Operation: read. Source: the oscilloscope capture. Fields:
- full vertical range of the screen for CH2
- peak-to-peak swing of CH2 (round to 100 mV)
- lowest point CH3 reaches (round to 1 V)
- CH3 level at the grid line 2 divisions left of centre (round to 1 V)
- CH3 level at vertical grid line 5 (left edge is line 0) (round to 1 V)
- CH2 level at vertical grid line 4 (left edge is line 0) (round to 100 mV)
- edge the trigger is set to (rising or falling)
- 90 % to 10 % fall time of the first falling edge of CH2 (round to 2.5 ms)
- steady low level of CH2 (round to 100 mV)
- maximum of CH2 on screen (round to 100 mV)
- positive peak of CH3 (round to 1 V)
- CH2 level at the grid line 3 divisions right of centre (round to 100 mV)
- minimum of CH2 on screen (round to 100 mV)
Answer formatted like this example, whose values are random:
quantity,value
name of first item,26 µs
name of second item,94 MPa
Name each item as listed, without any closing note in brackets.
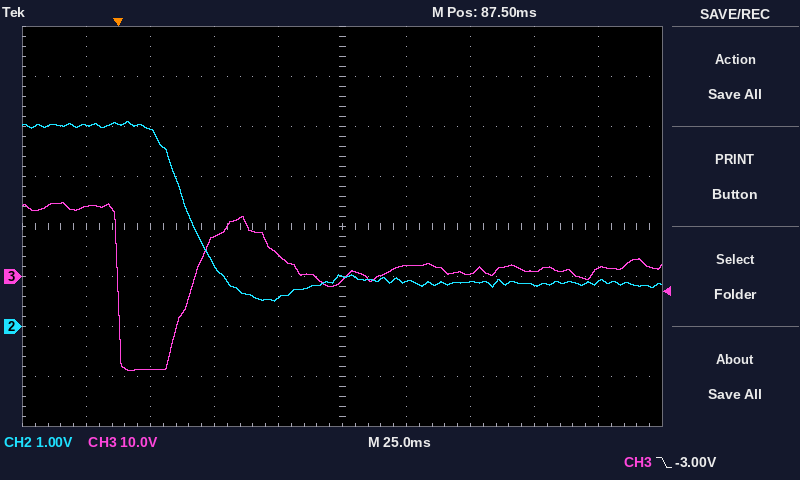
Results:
quantity,value
full vertical range of the screen for CH2,8 V
peak-to-peak swing of CH2,3.6 V
lowest point CH3 reaches,-19 V
CH3 level at the grid line 2 divisions left of centre,8 V
CH3 level at vertical grid line 5 (left edge is line 0),-1 V
CH2 level at vertical grid line 4 (left edge is line 0),600 mV
edge the trigger is set to,falling
90 % to 10 % fall time of the first falling edge of CH2,22.5 ms
steady low level of CH2,900 mV
maximum of CH2 on screen,4.1 V
positive peak of CH3,15 V
CH2 level at the grid line 3 divisions right of centre,800 mV
minimum of CH2 on screen,500 mV
